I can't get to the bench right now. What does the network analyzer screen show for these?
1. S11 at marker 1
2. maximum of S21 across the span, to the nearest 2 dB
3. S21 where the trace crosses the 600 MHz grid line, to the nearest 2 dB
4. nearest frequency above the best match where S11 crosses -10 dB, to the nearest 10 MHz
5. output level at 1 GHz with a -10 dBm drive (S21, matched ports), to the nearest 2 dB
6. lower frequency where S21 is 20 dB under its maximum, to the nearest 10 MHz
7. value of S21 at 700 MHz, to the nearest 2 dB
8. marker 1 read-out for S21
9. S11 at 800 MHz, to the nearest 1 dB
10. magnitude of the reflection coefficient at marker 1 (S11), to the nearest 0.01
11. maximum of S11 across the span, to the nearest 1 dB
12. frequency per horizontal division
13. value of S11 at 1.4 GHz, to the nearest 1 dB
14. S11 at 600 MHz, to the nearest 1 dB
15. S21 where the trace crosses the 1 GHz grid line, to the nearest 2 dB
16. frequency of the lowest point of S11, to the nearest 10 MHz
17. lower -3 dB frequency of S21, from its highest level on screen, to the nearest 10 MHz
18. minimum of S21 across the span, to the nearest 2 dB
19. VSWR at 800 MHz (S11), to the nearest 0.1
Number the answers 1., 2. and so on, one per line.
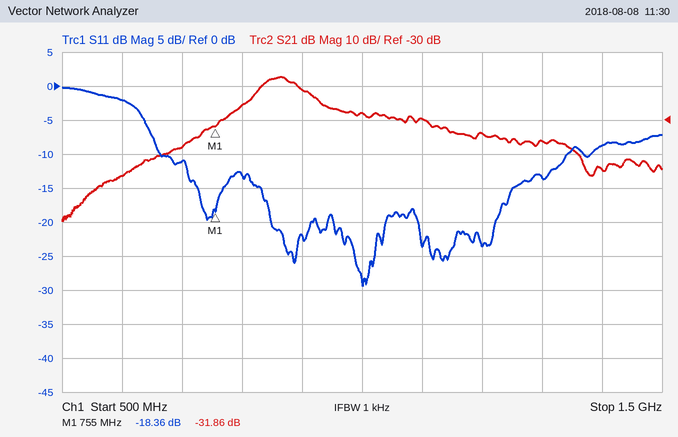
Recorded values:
1. -18.36 dB
2. -18 dB
3. -46 dB
4. 1.34 GHz
5. -38 dBm
6. 700 MHz
7. -38 dB
8. -31.86 dB
9. -13 dB
10. 0.12
11. 0 dB
12. 100 MHz
13. -9 dB
14. -2 dB
15. -28 dB
16. 1.00 GHz
17. 830 MHz
18. -60 dB
19. 1.6
